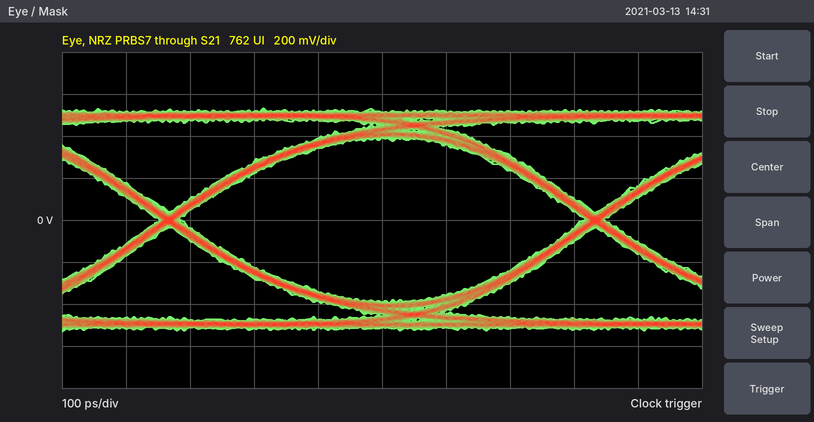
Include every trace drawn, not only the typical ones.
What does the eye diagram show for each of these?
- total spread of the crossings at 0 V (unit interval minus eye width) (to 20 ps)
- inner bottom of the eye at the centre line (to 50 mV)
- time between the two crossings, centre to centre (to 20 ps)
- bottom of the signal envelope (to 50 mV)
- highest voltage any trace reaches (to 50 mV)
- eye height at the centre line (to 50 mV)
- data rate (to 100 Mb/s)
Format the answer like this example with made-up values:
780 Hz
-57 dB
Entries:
40 ps
-400 mV
660 ps
-550 mV
550 mV
800 mV
1.5 Gb/s
